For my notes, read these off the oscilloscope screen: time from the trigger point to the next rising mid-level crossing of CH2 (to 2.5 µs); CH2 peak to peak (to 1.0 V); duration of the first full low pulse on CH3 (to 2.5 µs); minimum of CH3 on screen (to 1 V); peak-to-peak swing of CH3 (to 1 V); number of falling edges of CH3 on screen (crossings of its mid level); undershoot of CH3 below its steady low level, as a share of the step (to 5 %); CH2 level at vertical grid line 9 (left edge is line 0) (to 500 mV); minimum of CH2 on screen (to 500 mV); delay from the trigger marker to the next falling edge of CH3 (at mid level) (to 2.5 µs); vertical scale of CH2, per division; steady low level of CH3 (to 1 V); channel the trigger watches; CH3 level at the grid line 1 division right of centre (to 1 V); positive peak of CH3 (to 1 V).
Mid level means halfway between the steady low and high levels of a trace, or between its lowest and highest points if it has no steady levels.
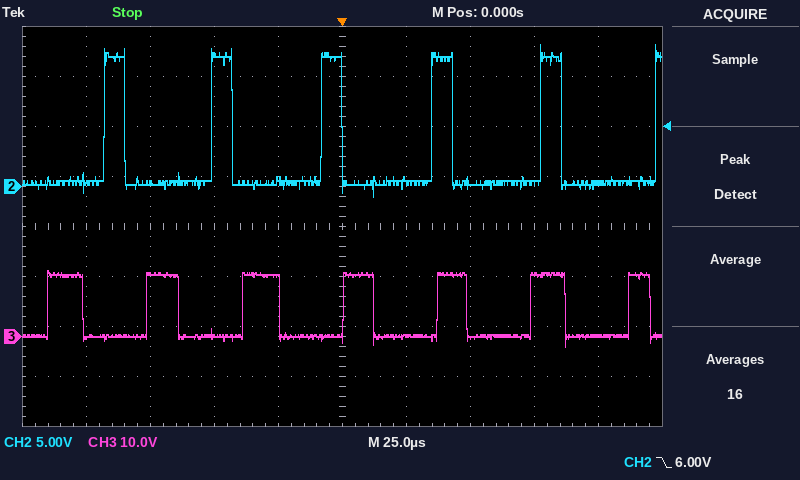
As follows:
35.0 µs
15.0 V
25.0 µs
-2 V
15 V
7
20 %
500 mV
-1.0 V
12.5 µs
5 V
0 V
CH2
0 V
13 V
